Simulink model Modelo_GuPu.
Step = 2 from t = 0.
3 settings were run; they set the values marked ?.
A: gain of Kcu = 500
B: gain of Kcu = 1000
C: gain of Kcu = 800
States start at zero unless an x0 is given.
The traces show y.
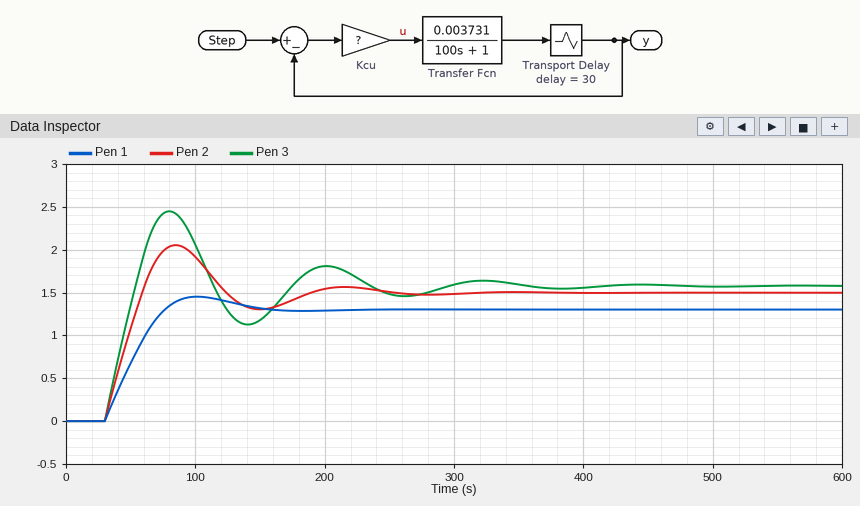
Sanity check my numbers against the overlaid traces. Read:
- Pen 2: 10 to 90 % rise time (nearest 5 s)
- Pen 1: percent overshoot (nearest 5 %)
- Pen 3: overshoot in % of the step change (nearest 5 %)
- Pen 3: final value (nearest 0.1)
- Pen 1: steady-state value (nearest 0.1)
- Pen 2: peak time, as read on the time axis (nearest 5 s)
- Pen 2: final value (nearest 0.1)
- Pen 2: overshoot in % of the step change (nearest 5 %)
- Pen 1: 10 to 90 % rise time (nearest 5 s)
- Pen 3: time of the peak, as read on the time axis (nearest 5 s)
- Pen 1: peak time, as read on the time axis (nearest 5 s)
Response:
25 s
10 %
55 %
1.6
1.3
85 s
1.5
35 %
35 s
80 s
100 s
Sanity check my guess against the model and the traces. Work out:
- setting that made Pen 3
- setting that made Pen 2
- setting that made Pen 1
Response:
B
C
A
